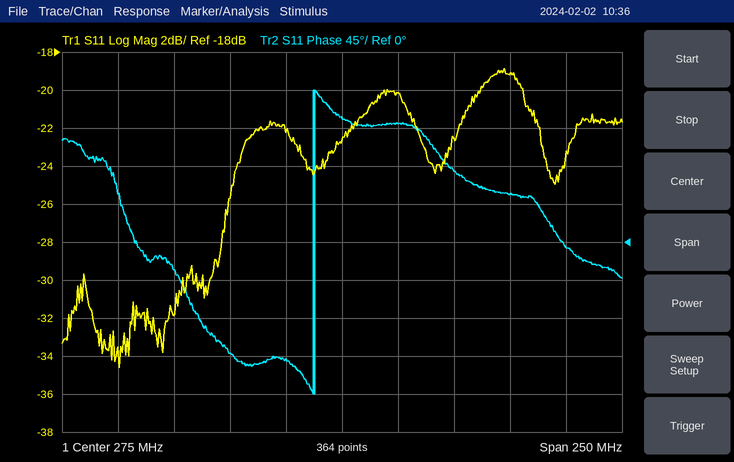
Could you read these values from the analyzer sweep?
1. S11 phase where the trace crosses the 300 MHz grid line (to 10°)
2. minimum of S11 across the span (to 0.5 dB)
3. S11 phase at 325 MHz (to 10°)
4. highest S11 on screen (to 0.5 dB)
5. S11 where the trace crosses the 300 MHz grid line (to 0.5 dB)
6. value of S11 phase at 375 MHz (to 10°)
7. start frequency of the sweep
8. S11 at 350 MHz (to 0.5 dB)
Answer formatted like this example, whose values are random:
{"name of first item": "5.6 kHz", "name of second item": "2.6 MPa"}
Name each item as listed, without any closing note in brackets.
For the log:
{"S11 phase where the trace crosses the 300 MHz grid line": "140°", "minimum of S11 across the span": "-34.5 dB", "S11 phase at 325 MHz": "80°", "highest S11 on screen": "-19.0 dB", "S11 where the trace crosses the 300 MHz grid line": "-20.0 dB", "value of S11 phase at 375 MHz": "-10°", "start frequency of the sweep": "150 MHz", "S11 at 350 MHz": "-19.0 dB"}
